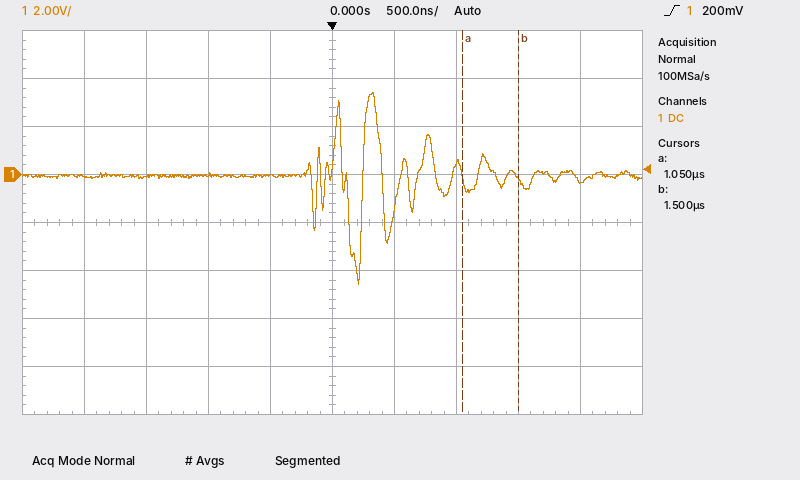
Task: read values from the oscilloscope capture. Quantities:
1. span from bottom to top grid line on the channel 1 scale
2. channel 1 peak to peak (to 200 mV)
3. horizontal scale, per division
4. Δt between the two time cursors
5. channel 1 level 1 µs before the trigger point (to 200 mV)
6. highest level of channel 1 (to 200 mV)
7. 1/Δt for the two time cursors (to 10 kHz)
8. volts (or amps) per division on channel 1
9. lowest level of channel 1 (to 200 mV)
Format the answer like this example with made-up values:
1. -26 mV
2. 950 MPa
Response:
1. 16 V
2. 8.0 V
3. 500 ns
4. 450 ns
5. 0.0 V
6. 3.4 V
7. 2.22 MHz
8. 2 V
9. -4.6 V
